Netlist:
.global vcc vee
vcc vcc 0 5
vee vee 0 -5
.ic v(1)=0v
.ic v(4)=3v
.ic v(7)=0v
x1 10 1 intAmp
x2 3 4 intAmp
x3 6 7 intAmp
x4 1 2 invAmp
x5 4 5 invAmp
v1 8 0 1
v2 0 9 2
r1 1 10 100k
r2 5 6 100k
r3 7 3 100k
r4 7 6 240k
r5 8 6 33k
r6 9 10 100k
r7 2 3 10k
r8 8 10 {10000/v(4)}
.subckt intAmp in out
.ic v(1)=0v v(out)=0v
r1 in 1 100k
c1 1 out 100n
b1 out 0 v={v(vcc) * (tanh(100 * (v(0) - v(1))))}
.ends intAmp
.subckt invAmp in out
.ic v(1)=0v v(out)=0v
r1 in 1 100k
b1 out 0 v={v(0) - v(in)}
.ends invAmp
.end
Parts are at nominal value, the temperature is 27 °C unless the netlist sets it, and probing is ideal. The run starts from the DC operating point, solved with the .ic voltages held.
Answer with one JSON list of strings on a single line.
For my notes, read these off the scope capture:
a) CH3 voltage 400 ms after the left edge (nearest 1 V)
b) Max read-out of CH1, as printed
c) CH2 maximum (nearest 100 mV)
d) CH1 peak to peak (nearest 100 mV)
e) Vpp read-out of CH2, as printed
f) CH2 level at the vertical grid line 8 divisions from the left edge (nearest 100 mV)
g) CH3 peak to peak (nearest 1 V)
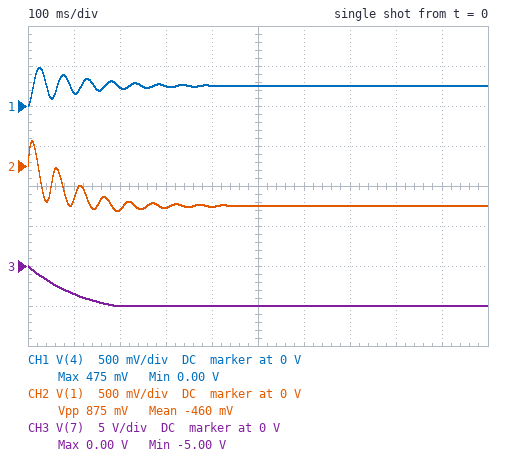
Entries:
["-5 V", "475 mV", "300 mV", "500 mV", "875 mV", "-500 mV", "5 V"]
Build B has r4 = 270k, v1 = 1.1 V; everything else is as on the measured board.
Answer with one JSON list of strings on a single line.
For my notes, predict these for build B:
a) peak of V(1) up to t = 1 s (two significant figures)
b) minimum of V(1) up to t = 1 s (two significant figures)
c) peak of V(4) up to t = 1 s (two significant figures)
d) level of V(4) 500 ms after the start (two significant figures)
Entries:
["300 mV", "-600 mV", "430 mV", "230 mV"]
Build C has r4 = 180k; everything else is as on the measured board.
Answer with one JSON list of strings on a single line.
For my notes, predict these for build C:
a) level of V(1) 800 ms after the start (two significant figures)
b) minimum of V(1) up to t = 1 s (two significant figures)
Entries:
["-480 mV", "-490 mV"]
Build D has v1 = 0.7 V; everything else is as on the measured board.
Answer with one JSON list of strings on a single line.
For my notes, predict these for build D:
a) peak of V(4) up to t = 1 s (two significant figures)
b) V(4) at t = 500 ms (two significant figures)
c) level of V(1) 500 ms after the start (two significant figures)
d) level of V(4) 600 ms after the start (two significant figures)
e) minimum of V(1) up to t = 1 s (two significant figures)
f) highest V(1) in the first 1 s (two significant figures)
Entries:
["670 mV", "350 mV", "-410 mV", "340 mV", "-430 mV", "360 mV"]
